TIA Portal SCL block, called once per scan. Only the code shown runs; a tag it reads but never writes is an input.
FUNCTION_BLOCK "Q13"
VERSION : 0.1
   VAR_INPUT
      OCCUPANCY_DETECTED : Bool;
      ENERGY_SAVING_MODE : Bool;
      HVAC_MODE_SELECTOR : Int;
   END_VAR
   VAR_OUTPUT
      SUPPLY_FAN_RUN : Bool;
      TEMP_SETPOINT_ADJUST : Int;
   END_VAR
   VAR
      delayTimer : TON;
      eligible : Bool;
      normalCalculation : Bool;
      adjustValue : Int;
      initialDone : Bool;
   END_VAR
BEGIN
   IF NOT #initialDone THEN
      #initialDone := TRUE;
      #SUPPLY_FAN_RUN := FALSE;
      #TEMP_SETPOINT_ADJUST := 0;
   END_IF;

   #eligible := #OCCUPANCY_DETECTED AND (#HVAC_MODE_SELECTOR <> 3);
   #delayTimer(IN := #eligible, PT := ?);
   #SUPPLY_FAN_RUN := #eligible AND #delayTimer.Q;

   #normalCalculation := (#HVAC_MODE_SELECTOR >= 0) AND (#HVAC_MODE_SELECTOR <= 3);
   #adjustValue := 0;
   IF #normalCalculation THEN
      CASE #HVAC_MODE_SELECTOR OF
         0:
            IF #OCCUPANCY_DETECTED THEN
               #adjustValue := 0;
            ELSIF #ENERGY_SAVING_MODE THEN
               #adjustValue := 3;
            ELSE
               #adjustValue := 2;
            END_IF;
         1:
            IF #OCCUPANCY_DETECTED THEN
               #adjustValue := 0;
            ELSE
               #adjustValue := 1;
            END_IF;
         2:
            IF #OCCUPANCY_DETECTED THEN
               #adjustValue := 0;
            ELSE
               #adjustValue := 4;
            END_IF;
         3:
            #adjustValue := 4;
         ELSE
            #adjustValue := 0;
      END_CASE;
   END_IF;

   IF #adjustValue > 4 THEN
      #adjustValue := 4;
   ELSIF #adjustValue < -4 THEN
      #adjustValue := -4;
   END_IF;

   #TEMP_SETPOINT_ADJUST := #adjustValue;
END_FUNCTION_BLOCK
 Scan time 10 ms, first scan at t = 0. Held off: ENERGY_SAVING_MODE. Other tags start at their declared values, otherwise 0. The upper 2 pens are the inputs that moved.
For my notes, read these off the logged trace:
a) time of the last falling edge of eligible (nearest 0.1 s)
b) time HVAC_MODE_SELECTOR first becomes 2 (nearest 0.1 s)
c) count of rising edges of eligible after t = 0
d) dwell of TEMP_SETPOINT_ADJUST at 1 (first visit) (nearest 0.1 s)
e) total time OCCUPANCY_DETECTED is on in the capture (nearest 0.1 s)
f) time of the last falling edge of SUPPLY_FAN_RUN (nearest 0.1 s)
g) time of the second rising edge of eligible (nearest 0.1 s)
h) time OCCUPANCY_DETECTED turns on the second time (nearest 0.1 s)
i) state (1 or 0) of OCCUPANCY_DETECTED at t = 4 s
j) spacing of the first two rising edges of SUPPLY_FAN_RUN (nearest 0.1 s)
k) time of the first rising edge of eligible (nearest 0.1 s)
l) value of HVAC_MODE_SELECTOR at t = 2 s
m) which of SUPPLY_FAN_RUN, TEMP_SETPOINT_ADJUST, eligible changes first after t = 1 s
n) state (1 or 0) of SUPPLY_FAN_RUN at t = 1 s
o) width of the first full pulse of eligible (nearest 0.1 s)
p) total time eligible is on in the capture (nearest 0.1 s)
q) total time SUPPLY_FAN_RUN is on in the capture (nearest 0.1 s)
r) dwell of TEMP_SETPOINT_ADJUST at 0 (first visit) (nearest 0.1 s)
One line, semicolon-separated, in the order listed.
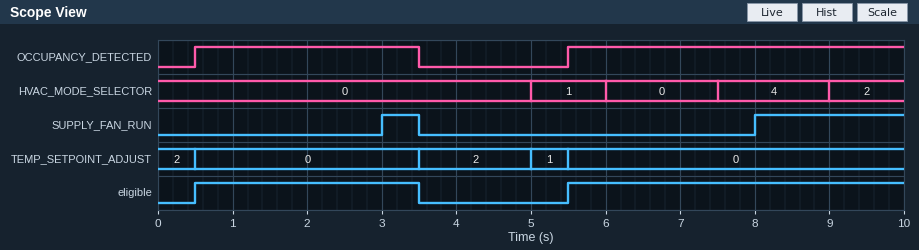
3.5 s; 9.0 s; 2; 0.5 s; 7.5 s; 3.5 s; 5.5 s; 5.5 s; 0; 5.0 s; 0.5 s; 0; SUPPLY_FAN_RUN; 0; 3.0 s; 7.5 s; 2.5 s; 3.0 s
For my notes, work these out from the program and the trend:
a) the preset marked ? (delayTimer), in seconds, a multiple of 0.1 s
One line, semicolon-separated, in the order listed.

2.5 s
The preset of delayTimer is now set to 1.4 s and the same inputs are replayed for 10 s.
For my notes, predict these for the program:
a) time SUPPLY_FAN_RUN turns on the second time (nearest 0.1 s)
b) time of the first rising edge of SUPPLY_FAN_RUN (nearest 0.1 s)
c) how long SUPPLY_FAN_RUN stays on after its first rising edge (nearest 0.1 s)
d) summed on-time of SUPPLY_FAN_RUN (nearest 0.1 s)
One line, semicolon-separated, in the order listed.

6.9 s; 1.9 s; 1.6 s; 4.7 s
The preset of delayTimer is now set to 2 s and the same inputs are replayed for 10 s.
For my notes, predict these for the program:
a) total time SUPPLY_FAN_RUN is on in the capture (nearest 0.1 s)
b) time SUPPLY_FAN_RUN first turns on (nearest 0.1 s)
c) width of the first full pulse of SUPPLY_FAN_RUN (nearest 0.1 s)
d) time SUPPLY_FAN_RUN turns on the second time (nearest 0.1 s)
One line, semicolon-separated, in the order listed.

3.5 s; 2.5 s; 1.0 s; 7.5 s
